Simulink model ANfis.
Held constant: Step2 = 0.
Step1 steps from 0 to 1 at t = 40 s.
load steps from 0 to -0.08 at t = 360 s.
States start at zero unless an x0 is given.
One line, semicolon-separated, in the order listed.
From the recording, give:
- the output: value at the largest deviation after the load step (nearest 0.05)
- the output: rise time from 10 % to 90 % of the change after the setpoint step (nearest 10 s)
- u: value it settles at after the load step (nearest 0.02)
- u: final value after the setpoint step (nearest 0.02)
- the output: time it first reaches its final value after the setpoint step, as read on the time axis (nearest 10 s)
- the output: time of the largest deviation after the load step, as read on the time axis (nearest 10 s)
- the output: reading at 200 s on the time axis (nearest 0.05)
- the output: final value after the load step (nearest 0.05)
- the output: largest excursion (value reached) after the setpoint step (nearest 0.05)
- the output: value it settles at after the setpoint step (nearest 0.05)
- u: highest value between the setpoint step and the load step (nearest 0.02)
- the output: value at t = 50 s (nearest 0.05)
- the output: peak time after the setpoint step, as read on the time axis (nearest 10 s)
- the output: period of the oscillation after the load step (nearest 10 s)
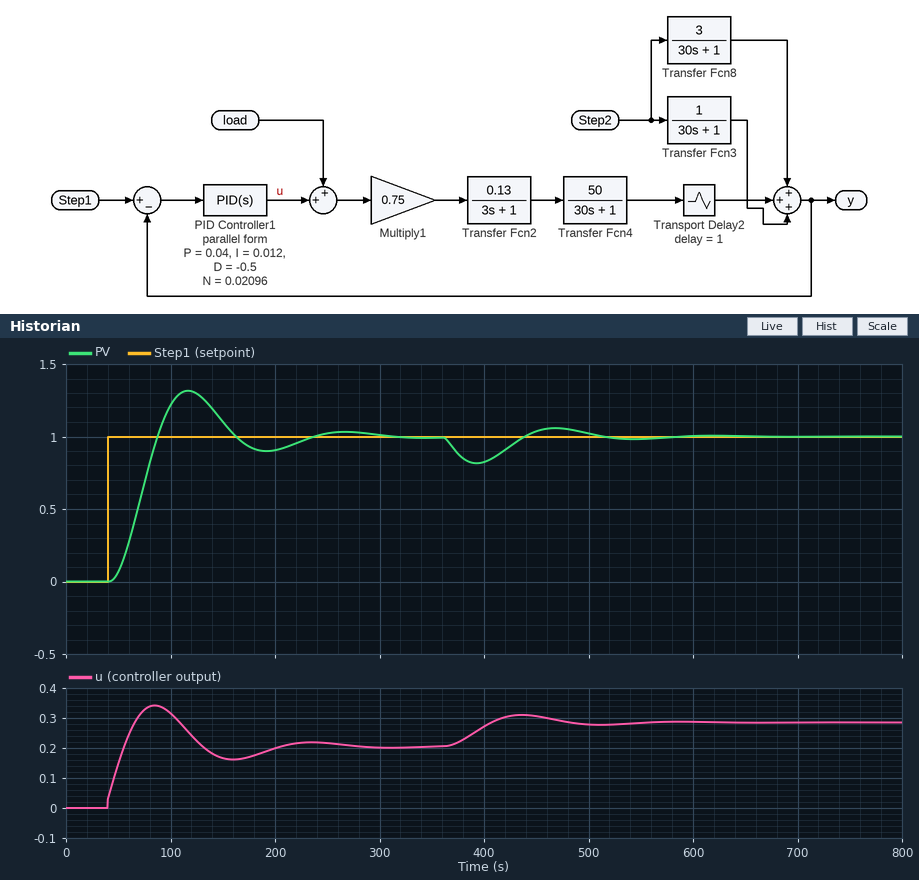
0.80; 30 s; 0.28; 0.20; 90 s; 390 s; 0.90; 1.00; 1.30; 1.00; 0.34; 0.05; 120 s; 150 s
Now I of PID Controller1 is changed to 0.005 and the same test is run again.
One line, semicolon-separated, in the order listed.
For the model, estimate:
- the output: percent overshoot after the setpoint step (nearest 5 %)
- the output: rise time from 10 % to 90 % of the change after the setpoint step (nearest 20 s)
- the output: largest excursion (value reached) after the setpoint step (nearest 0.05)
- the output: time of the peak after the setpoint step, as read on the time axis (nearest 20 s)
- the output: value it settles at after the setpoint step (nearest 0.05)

10 %; 60 s; 1.10; 180 s; 1.00
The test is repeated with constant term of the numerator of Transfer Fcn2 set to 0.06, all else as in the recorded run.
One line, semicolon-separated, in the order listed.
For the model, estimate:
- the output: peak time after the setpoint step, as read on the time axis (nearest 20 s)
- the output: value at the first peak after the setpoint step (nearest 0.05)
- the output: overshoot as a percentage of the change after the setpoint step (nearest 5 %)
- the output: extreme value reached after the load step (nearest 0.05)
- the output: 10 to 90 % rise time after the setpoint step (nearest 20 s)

160 s; 1.15; 15 %; 0.90; 60 s
